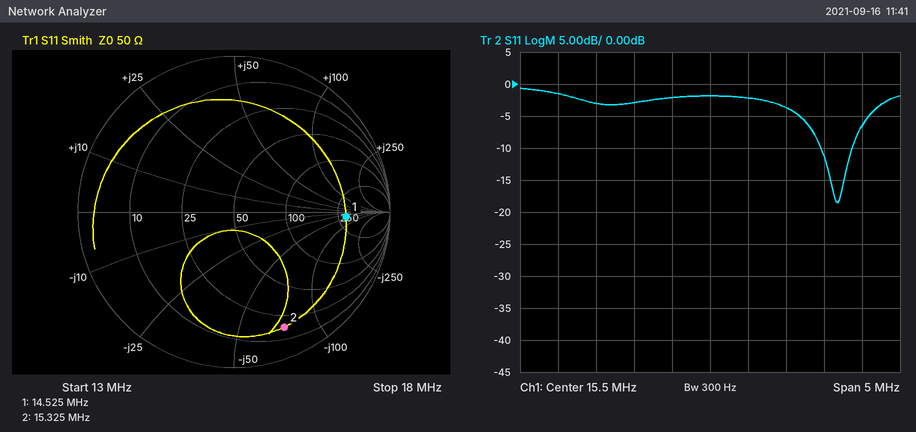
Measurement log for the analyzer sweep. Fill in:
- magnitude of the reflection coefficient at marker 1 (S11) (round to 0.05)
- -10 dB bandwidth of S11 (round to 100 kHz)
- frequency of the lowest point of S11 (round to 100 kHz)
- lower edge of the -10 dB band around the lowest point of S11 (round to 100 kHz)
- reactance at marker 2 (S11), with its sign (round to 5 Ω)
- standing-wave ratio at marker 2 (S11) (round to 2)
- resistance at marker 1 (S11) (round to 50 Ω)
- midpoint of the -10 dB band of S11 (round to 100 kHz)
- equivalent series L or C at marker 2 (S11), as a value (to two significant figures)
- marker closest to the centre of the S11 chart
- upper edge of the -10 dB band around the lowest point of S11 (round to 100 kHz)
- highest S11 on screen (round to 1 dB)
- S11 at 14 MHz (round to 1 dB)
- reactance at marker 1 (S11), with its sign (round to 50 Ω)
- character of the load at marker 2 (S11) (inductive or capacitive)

0.70
400 kHz
17.2 MHz
17.0 MHz
-75 Ω
10
300 Ω
17.2 MHz
140 pF
marker 1
17.4 MHz
-1 dB
-3 dB
-50 Ω
capacitive
